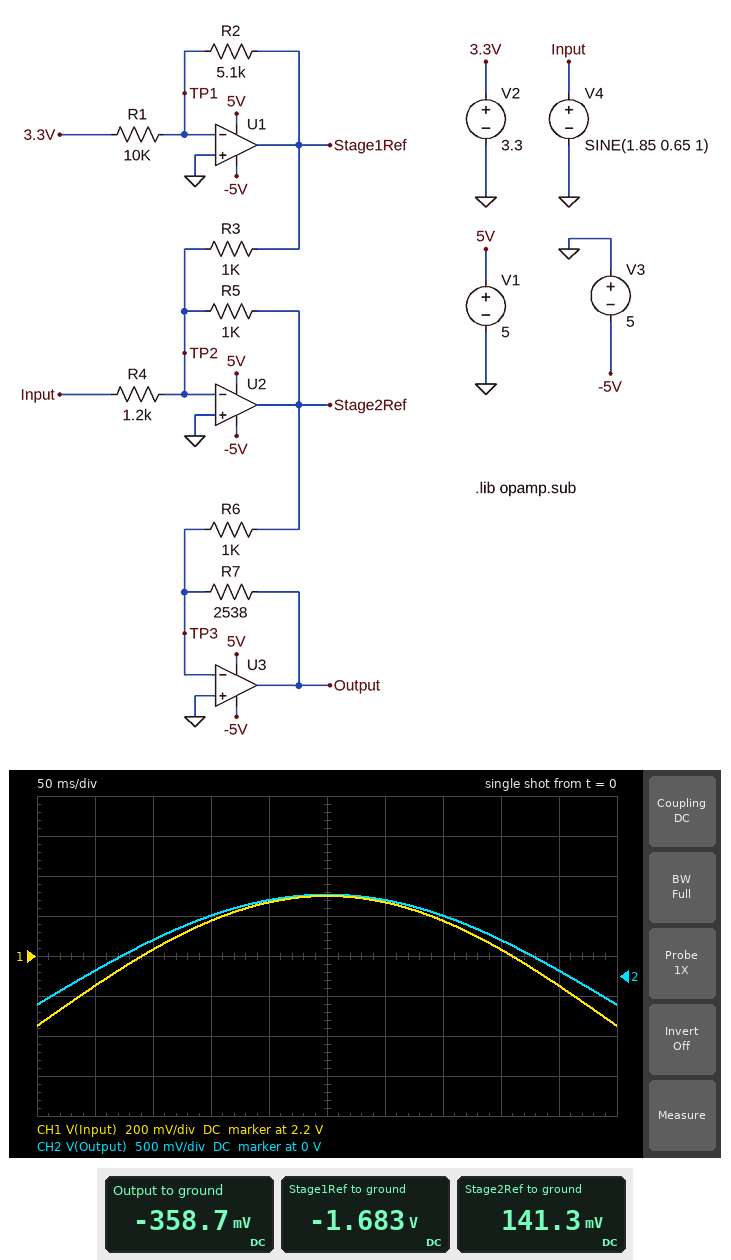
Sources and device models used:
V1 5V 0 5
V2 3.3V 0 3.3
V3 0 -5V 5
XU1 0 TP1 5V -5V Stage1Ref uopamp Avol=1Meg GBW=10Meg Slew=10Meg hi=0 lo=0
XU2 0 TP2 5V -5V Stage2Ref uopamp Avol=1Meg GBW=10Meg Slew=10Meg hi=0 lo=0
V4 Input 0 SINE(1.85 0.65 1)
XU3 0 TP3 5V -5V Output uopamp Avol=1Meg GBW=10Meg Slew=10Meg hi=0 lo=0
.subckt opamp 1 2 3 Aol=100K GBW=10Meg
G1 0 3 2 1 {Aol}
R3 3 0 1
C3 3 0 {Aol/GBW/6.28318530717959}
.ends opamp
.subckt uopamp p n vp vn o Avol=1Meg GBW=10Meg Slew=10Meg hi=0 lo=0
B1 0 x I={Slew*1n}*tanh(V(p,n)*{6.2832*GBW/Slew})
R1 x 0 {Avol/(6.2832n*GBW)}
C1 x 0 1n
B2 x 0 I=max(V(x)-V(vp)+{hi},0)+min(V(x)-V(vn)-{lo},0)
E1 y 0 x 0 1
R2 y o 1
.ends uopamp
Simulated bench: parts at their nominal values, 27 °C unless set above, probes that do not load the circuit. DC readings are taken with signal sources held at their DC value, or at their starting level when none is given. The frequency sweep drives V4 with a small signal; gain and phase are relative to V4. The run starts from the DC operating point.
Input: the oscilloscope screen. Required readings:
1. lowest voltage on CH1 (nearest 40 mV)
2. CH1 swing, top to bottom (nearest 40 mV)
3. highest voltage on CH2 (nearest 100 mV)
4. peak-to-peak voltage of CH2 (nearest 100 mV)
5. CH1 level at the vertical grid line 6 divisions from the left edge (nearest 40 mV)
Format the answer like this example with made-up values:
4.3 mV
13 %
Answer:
1.84 V
640 mV
1.0 V
1.4 V
2.48 V
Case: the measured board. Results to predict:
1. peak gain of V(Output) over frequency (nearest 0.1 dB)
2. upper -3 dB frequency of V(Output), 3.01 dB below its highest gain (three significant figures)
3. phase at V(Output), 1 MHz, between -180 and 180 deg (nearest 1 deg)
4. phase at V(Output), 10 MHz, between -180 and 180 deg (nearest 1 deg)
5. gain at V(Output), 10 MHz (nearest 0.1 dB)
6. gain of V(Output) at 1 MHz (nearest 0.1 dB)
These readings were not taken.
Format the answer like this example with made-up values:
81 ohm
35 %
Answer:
6.5 dB
2.01 MHz
-35 deg
-145 deg
-14.4 dB
5.7 dB
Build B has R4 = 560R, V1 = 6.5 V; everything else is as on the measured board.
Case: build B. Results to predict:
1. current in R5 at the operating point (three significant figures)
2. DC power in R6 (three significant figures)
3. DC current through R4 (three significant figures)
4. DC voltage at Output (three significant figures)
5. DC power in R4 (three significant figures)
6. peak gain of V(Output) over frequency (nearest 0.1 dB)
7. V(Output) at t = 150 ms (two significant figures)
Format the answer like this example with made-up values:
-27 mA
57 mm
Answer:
1.62 mA
2.63 mW
3.30 mA
4.11 V
6.11 mW
13.1 dB
6.5 V
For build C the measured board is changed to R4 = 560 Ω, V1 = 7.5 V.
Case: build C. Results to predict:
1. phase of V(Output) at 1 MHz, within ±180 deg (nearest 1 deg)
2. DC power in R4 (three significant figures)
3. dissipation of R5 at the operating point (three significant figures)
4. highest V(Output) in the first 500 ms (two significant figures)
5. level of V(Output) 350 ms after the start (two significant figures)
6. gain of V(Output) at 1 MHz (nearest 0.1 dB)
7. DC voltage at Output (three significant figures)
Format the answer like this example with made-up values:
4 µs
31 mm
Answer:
-40 deg
6.11 mW
2.63 mW
7.1 V
6.5 V
12.0 dB
4.11 V
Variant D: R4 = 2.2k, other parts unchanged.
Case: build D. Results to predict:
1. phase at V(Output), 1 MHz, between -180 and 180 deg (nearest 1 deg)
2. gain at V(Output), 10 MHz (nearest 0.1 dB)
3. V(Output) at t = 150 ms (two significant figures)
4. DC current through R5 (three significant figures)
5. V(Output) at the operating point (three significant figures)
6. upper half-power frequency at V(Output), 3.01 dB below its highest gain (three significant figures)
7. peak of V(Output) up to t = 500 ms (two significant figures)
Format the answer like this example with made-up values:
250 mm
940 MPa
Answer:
-33 deg
-18.5 dB
-1.5 V
842 µA
-2.14 V
2.13 MHz
-1.4 V
